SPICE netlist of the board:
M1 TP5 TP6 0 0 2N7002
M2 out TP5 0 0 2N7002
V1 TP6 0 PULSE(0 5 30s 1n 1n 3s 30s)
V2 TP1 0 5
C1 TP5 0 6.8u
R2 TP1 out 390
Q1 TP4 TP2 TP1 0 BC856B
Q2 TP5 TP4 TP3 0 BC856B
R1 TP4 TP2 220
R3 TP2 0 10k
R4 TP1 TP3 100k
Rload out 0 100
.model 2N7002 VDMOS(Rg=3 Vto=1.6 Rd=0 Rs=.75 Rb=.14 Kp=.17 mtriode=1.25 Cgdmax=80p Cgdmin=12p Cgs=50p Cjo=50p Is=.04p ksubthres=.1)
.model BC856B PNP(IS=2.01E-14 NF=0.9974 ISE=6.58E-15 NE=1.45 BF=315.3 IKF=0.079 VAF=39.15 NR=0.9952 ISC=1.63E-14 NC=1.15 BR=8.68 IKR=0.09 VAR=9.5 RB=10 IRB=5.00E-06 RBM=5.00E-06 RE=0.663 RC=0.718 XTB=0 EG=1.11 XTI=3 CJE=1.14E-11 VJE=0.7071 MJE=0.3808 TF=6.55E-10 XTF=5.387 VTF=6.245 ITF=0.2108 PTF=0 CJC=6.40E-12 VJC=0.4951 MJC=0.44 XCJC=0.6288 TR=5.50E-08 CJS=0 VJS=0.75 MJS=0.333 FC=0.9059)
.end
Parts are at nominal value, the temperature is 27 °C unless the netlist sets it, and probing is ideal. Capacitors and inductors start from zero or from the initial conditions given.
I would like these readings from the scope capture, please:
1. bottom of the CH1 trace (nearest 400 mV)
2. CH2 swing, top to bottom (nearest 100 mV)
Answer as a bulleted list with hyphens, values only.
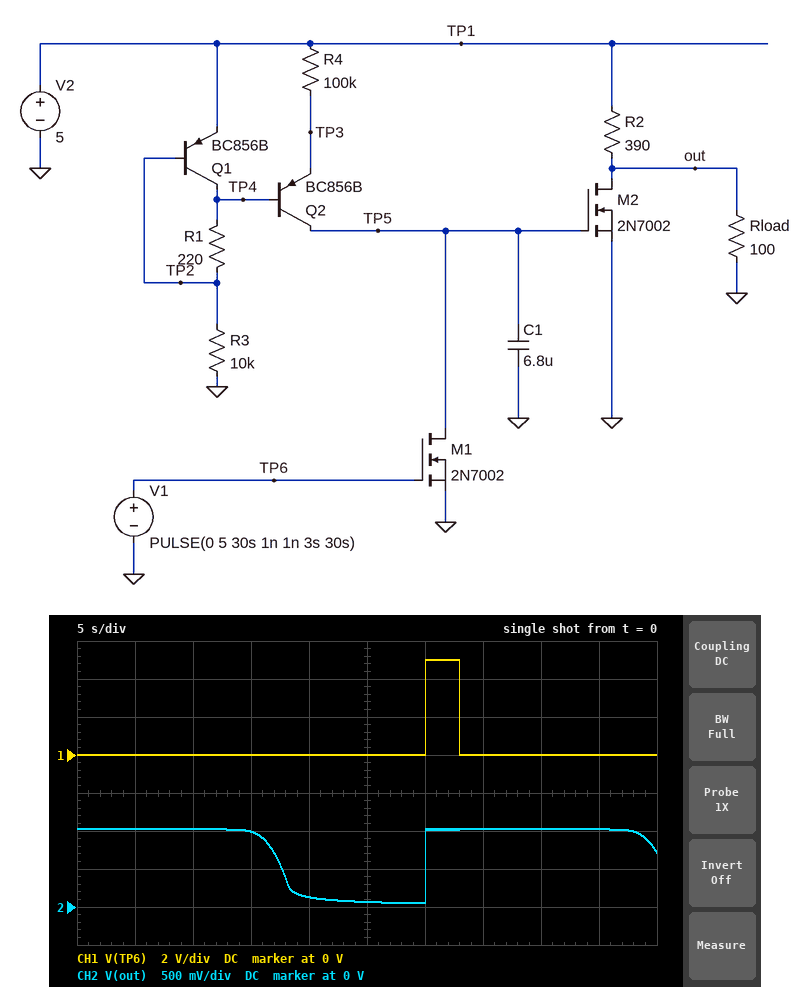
- 0 V
- 1.0 V
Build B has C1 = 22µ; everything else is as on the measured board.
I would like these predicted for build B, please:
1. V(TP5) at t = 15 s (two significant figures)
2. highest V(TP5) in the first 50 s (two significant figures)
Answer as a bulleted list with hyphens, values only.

- 490 mV
- 990 mV
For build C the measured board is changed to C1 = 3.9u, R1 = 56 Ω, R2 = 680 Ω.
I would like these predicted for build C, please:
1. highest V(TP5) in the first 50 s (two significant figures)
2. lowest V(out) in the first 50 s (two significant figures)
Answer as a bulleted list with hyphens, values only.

- 4.9 V
- 16 mV
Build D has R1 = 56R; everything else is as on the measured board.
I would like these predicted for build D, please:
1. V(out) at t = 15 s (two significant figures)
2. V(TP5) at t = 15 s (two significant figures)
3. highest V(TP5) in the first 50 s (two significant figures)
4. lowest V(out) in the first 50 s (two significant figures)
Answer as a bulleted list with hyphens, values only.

- 57 mV
- 2.8 V
- 4.9 V
- 27 mV
